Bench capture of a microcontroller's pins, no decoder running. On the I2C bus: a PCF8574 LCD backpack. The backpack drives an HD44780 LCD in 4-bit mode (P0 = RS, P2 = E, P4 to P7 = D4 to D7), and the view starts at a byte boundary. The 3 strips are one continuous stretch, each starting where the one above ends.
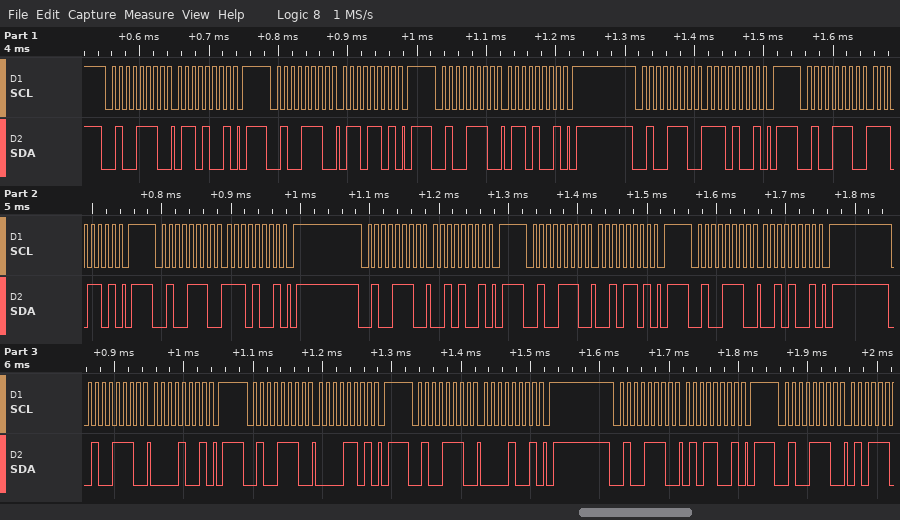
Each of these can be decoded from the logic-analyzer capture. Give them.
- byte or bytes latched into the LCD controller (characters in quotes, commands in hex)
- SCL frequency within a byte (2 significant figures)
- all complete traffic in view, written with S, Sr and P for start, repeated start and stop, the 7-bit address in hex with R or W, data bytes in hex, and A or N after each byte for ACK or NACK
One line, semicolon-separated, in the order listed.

'n' ' '; 100 kHz; S 27W A 69 A P S 27W A 6D A P S 27W A 69 A P S 27W A E9 A P S 27W A ED A P S 27W A E9 A P S 27W A 29 A P S 27W A 2D A P S 27W A 29 A P S 27W A 09 A P S 27W A 0D A P S 27W A 09 A P S 27W A 59 A P S 27W A
